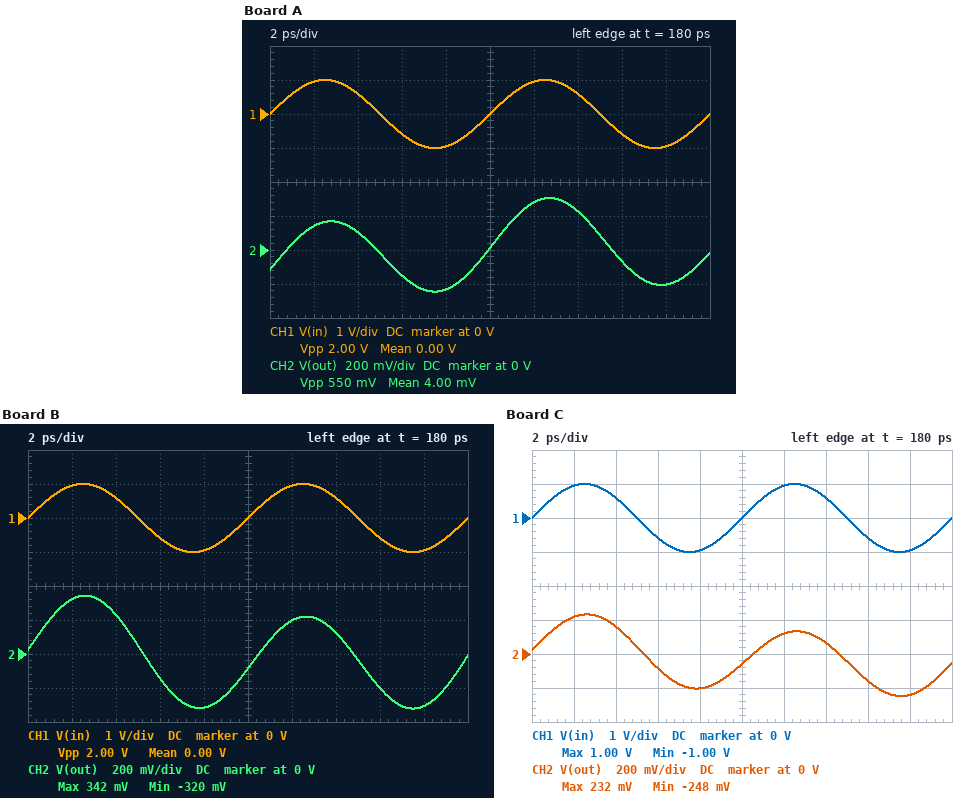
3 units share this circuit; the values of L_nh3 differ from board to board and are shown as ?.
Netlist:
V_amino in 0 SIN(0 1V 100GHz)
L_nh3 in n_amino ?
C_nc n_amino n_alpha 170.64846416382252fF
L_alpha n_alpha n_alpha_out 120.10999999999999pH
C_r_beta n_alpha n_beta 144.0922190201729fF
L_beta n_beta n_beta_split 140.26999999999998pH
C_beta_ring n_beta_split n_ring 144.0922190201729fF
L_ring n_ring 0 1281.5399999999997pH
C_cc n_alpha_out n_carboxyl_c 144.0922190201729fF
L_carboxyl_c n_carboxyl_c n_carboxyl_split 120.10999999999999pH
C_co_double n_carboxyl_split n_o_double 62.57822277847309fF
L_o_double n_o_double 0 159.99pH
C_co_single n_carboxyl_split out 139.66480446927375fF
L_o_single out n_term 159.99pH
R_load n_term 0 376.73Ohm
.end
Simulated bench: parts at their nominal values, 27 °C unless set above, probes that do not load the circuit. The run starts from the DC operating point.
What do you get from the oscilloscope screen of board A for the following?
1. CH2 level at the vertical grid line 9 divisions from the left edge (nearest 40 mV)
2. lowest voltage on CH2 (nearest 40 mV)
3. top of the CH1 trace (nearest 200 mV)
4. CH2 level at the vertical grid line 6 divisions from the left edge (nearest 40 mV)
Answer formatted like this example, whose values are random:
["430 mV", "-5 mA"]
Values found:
["-200 mV", "-240 mV", "1.0 V", "280 mV"]
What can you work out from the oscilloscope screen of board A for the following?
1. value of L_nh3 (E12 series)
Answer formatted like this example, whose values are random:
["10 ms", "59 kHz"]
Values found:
["120 pH"]
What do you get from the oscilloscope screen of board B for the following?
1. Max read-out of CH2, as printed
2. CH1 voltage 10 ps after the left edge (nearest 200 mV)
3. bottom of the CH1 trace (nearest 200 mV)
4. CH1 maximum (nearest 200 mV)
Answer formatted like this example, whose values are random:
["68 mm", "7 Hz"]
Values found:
["342 mV", "0 V", "-1.0 V", "1.0 V"]
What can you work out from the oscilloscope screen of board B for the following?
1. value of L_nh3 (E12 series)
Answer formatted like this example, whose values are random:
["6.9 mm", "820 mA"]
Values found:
["56 pH"]
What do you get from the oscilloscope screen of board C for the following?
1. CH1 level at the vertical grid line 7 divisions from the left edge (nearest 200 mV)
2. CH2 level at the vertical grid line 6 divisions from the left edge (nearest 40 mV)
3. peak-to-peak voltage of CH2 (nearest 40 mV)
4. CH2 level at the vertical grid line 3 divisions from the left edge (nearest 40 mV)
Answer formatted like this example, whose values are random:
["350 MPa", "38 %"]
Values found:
["600 mV", "120 mV", "480 mV", "-80 mV"]
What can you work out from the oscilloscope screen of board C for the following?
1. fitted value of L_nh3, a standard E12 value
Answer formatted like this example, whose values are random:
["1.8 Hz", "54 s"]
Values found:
["220 pH"]
